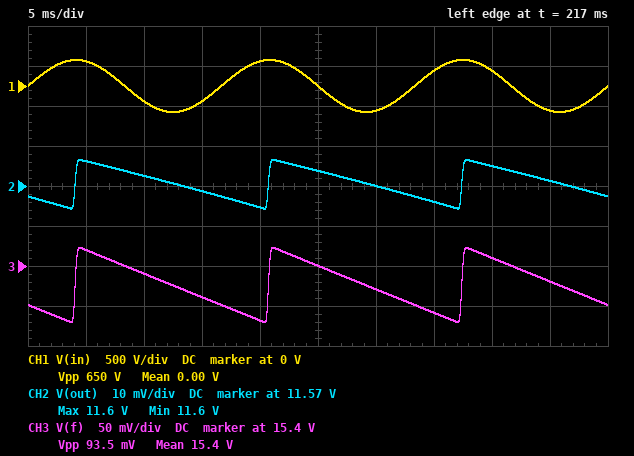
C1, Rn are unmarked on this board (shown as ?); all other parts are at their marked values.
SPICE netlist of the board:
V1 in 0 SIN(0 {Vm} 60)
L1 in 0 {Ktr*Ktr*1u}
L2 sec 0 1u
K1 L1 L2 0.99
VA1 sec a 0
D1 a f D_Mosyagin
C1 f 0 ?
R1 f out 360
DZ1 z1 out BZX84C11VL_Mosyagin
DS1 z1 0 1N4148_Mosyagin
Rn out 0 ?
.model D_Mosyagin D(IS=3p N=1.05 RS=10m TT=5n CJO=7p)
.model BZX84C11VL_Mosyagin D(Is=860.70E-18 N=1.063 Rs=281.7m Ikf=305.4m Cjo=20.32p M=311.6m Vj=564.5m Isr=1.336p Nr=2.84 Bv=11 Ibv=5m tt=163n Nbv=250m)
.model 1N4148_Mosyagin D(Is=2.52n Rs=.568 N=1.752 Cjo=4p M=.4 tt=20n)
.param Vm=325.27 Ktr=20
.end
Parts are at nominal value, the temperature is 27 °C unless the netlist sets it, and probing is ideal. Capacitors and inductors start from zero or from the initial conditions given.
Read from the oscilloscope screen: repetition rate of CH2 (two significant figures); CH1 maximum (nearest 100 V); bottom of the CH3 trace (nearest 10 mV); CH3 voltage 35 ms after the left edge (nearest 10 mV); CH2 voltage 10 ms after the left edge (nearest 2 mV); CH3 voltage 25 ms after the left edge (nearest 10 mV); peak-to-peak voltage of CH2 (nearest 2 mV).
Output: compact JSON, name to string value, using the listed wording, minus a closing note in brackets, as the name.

{"repetition rate of CH2": "60 Hz", "CH1 maximum": "300 V", "bottom of the CH3 trace": "15.33 V", "CH3 voltage 35 ms after the left edge": "15.34 V", "CH2 voltage 10 ms after the left edge": "11.572 V", "CH3 voltage 25 ms after the left edge": "15.40 V", "peak-to-peak voltage of CH2": "12 mV"}
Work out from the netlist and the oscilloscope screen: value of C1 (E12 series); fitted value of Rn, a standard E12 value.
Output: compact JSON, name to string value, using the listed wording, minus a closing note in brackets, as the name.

{"value of C1": "1.8 mF", "fitted value of Rn, a standard E12 value": "1.2 kΩ"}
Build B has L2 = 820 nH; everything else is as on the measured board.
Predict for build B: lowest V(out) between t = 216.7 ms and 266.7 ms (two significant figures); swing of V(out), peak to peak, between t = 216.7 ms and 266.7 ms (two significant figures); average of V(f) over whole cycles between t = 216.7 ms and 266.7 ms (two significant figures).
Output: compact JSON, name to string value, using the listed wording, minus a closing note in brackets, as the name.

{"lowest V(out) between t = 216.7 ms and 266.7 ms": "11 V", "swing of V(out), peak to peak, between t = 216.7 ms and 266.7 ms": "60 mV", "average of V(f) over whole cycles between t = 216.7 ms and 266.7 ms": "14 V"}
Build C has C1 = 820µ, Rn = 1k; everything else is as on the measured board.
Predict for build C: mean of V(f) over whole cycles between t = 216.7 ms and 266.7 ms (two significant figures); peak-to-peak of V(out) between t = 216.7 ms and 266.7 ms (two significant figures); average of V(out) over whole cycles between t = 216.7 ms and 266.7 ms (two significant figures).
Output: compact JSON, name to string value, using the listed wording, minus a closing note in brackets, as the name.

{"mean of V(f) over whole cycles between t = 216.7 ms and 266.7 ms": "15 V", "peak-to-peak of V(out) between t = 216.7 ms and 266.7 ms": "160 mV", "average of V(out) over whole cycles between t = 216.7 ms and 266.7 ms": "11 V"}
